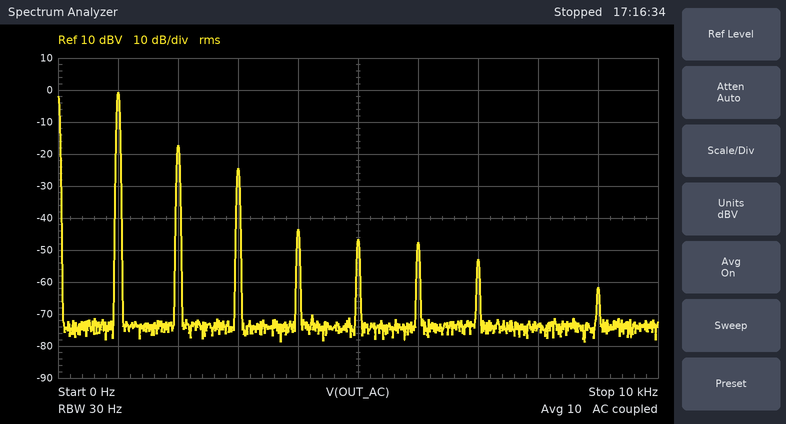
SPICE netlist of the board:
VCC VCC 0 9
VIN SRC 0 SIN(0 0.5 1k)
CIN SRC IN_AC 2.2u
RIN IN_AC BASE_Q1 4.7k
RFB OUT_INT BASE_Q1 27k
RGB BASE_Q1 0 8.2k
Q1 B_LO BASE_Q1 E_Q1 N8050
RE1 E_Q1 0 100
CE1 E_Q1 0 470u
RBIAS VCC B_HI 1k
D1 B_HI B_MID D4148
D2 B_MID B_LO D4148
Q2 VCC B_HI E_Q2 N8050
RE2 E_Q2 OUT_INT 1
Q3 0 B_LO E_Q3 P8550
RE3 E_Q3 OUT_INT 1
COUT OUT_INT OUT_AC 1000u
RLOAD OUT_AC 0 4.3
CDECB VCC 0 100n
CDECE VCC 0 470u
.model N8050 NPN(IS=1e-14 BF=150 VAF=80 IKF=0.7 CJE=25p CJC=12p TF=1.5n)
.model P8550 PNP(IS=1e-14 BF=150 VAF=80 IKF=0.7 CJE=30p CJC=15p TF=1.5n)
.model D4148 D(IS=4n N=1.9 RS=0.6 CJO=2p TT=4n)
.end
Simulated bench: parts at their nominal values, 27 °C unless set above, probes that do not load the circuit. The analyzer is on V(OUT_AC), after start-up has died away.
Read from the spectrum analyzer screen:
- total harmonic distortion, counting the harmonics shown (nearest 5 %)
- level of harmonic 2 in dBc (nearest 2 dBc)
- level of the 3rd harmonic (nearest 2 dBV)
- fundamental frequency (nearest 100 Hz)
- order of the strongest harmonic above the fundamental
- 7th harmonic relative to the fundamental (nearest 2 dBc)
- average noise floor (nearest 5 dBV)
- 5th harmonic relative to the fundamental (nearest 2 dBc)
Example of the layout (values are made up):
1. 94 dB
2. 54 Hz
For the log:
1. 15 %
2. -16 dBc
3. -24 dBV
4. 1.0 kHz
5. 2
6. -52 dBc
7. -75 dBV
8. -46 dBc
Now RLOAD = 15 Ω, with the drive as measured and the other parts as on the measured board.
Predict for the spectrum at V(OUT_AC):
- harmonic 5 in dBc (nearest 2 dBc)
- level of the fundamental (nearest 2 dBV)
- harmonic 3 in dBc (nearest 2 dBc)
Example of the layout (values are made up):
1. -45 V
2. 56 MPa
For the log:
1. -52 dBc
2. 2 dBV
3. -38 dBc
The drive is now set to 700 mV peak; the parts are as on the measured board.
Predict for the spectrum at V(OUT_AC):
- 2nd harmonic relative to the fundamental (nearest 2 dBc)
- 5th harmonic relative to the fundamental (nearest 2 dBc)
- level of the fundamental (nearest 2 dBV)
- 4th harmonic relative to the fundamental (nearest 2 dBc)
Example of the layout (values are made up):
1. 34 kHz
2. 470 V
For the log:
1. -12 dBc
2. -32 dBc
3. 0 dBV
4. -30 dBc
